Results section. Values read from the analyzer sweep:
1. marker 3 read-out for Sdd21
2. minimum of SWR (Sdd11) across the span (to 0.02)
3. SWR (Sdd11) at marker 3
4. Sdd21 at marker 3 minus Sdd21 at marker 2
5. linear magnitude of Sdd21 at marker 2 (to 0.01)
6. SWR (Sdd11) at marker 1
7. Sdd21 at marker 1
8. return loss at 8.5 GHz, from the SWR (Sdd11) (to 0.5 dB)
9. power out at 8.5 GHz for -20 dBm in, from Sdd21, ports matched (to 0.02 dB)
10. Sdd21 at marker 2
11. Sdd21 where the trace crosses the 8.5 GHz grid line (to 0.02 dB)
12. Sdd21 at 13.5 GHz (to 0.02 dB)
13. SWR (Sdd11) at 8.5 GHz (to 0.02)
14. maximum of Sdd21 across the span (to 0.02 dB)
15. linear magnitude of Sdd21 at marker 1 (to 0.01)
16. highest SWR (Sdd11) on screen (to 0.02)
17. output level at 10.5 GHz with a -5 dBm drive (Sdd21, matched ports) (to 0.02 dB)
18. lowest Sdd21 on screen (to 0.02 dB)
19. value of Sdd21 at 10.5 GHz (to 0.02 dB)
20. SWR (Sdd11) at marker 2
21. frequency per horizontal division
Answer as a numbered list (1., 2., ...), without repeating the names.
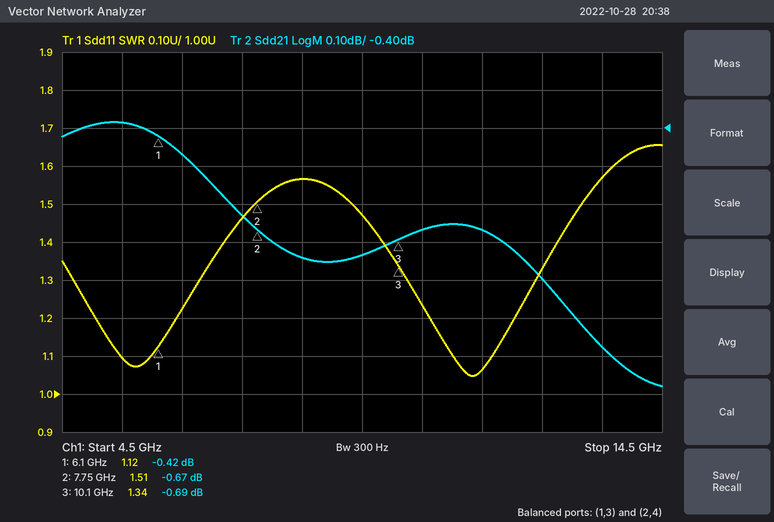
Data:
1. -0.69 dB
2. 1.04
3. 1.34
4. -0.02 dB
5. 0.93
6. 1.12
7. -0.42 dB
8. 13.0 dB
9. -20.74 dBm
10. -0.67 dB
11. -0.74 dB
12. -0.98 dB
13. 1.56
14. -0.38 dB
15. 0.95
16. 1.66
17. -5.66 dBm
18. -1.08 dB
19. -0.66 dB
20. 1.51
21. 1 GHz
